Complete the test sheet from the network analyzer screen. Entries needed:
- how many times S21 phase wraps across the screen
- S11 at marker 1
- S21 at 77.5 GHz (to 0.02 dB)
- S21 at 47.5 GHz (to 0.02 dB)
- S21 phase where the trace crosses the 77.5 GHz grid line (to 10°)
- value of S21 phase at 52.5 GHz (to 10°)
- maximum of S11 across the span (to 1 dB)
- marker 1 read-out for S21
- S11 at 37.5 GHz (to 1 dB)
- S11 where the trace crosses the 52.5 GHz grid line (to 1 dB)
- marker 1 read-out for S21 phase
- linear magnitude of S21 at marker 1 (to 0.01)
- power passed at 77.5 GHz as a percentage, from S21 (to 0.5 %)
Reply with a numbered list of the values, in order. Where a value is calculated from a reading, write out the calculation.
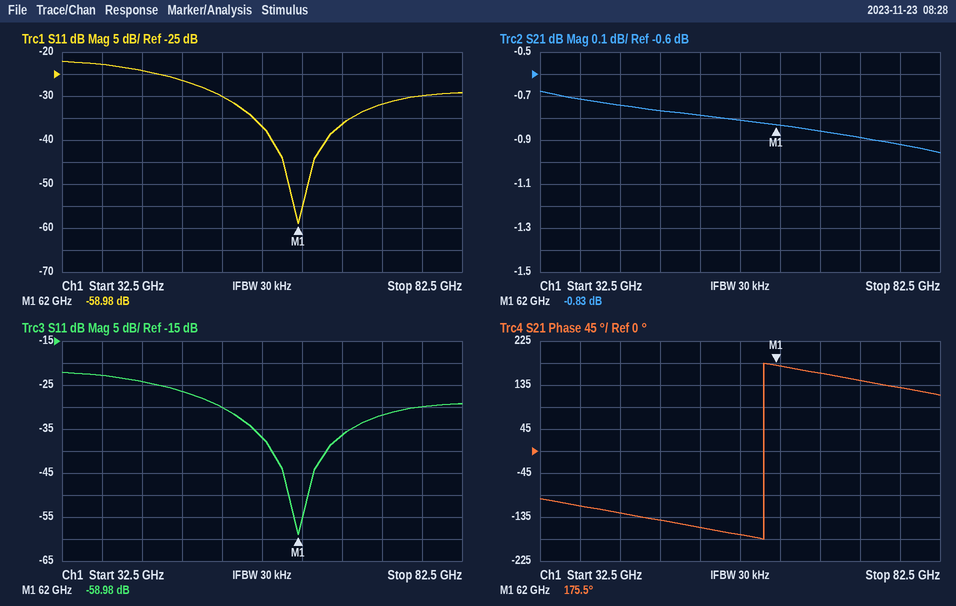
1. 1
2. -58.98 dB
3. -0.92 dB
4. -0.76 dB
5. 130°
6. -160°
7. -22 dB
8. -0.83 dB
9. -23 dB
10. -30 dB
11. 175.5°
12. 10^(-0.83/20) ≈ 0.91
13. 10^(-0.92/10) ≈ 80.9 %, so 81.0 % to the nearest 0.5 %
